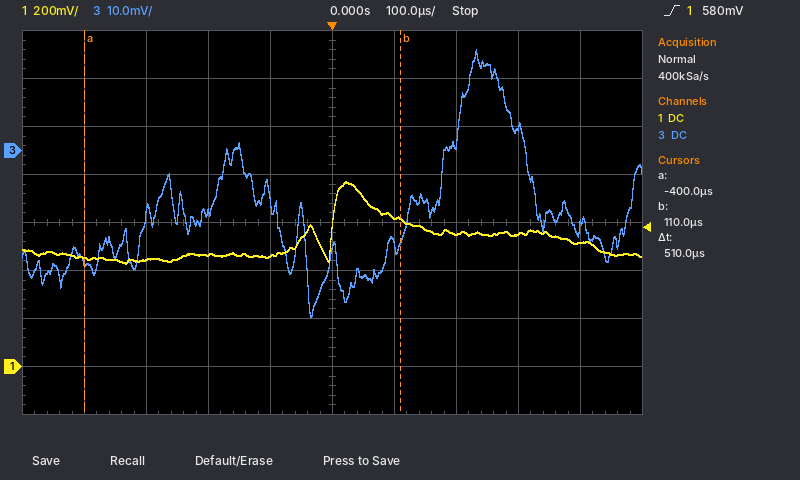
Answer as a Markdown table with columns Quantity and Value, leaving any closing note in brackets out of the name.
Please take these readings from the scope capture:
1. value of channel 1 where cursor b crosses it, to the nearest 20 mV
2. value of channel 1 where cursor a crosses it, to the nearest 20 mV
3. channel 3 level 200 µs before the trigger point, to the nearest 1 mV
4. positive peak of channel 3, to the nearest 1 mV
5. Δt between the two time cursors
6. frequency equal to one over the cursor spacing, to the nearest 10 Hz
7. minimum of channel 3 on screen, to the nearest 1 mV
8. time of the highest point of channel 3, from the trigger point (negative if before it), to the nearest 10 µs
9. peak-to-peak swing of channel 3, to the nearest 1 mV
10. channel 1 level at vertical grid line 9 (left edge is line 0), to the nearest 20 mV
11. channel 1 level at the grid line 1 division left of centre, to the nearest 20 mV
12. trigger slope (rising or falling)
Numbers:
| Quantity | Value |
|---|---|
| value of channel 1 where cursor b crosses it, to the nearest 20 mV | 620 mV |
| value of channel 1 where cursor a crosses it, to the nearest 20 mV | 460 mV |
| channel 3 level 200 µs before the trigger point, to the nearest 1 mV | -13 mV |
| positive peak of channel 3, to the nearest 1 mV | 21 mV |
| Δt between the two time cursors | 510 µs |
| frequency equal to one over the cursor spacing, to the nearest 10 Hz | 1.96 kHz |
| minimum of channel 3 on screen, to the nearest 1 mV | -35 mV |
| time of the highest point of channel 3, from the trigger point (negative if before it), to the nearest 10 µs | +230 µs |
| peak-to-peak swing of channel 3, to the nearest 1 mV | 56 mV |
| channel 1 level at vertical grid line 9 (left edge is line 0), to the nearest 20 mV | 520 mV |
| channel 1 level at the grid line 1 division left of centre, to the nearest 20 mV | 460 mV |
| trigger slope | rising |
